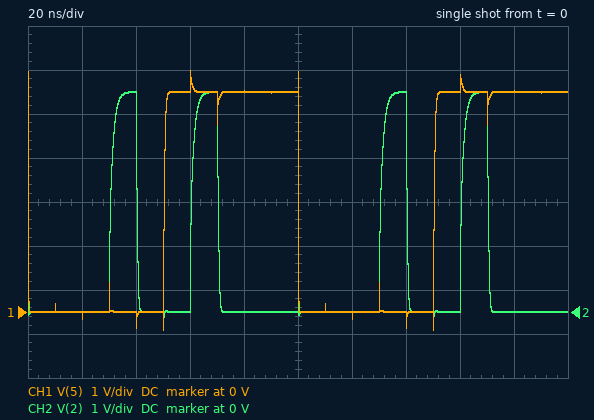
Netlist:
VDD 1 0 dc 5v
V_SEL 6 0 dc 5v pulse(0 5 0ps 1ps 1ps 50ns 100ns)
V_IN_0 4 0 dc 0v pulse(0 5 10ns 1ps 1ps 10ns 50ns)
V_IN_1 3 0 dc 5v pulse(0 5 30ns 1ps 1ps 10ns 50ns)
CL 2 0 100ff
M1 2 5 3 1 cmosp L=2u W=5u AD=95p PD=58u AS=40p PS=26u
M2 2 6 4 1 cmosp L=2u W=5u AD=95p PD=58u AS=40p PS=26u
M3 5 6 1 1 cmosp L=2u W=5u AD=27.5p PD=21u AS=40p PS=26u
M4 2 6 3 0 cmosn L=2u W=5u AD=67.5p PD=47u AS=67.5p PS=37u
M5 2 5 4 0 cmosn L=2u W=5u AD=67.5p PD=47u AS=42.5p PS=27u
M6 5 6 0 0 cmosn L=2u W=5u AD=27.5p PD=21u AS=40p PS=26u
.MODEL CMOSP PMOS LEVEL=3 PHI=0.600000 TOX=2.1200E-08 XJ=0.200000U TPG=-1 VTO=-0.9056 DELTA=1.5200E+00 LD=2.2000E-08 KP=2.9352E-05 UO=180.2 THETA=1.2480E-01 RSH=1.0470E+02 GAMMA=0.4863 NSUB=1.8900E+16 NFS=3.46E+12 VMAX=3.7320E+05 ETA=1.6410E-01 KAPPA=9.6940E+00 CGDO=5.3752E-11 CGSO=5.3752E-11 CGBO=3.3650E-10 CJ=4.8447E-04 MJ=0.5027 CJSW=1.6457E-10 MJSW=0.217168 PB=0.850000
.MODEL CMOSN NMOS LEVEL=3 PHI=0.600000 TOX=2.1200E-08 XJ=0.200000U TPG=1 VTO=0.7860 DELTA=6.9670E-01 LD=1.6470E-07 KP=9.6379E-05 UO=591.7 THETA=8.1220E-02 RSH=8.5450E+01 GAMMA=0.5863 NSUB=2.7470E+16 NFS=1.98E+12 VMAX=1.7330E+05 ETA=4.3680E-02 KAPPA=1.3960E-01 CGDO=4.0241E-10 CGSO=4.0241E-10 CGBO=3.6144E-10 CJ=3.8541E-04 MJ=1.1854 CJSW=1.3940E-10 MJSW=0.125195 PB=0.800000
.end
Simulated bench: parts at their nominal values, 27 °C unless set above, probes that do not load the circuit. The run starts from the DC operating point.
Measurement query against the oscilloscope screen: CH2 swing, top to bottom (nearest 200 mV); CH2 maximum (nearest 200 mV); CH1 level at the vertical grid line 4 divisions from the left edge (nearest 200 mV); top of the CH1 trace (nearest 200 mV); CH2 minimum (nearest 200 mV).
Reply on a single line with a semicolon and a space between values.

5.2 V; 5.0 V; 5.0 V; 5.4 V; -200 mV
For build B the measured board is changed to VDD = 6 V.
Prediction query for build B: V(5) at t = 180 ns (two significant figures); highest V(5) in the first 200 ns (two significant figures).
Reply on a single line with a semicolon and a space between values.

6.0 V; 6.5 V
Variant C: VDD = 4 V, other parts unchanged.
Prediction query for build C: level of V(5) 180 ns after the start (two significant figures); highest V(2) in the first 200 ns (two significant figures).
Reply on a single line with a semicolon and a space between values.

4.0 V; 4.5 V
